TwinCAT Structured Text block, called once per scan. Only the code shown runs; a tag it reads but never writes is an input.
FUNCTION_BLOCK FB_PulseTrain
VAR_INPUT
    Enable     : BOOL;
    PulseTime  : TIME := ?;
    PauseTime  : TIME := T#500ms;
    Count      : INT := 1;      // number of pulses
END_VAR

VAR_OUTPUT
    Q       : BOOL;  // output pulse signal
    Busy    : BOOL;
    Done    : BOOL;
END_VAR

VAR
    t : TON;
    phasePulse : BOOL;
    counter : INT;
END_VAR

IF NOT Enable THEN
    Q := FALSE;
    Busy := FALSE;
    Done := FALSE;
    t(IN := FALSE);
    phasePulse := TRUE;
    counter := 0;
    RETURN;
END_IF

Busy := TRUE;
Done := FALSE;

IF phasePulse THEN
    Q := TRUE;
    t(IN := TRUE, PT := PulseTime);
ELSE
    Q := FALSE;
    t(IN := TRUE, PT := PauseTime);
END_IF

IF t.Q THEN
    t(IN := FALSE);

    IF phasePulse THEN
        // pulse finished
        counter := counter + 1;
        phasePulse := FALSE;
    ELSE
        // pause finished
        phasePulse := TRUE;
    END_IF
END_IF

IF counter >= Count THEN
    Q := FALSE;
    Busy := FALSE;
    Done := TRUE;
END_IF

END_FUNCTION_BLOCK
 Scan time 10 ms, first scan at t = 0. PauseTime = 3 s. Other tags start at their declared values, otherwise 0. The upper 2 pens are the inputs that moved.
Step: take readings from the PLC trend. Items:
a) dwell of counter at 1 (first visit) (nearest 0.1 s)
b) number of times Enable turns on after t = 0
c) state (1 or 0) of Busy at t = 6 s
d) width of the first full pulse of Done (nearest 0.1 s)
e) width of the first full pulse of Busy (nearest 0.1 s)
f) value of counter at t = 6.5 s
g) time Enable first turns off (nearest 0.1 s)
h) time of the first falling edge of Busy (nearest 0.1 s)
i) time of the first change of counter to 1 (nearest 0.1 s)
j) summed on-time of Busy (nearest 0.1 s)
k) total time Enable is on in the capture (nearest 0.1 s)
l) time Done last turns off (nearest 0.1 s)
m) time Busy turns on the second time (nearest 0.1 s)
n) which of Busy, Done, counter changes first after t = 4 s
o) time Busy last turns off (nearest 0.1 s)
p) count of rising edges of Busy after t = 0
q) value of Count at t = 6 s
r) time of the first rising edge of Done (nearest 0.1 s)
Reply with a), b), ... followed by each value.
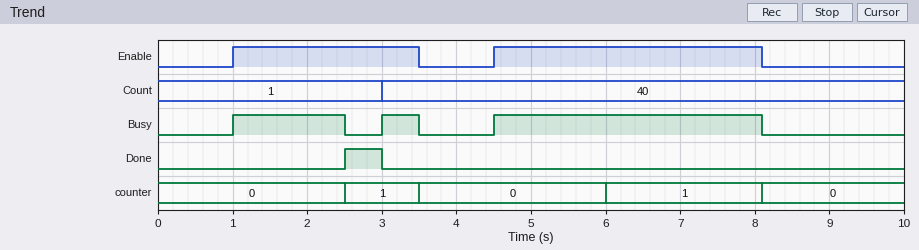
a) 1.0 s
b) 2
c) 1
d) 0.5 s
e) 1.5 s
f) 1
g) 3.5 s
h) 2.5 s
i) 2.5 s
j) 5.6 s
k) 6.1 s
l) 3.0 s
m) 3.0 s
n) Busy
o) 8.1 s
p) 3
q) 40
r) 2.5 s
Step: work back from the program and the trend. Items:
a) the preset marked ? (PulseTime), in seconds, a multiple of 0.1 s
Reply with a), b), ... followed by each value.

a) 1.5 s
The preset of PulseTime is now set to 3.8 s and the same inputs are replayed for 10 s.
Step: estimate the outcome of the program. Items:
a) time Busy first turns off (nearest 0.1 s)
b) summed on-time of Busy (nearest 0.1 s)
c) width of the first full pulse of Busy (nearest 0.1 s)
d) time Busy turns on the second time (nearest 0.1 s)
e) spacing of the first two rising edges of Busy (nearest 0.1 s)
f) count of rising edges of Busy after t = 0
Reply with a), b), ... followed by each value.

a) 3.5 s
b) 6.1 s
c) 2.5 s
d) 4.5 s
e) 3.5 s
f) 2
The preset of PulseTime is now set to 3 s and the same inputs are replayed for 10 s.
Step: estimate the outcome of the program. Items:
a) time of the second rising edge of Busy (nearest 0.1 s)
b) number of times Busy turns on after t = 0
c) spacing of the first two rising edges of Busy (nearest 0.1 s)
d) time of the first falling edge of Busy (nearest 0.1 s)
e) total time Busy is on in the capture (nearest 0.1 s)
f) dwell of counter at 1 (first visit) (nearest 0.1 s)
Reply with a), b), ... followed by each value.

a) 4.5 s
b) 2
c) 3.5 s
d) 3.5 s
e) 6.1 s
f) 0.6 s
